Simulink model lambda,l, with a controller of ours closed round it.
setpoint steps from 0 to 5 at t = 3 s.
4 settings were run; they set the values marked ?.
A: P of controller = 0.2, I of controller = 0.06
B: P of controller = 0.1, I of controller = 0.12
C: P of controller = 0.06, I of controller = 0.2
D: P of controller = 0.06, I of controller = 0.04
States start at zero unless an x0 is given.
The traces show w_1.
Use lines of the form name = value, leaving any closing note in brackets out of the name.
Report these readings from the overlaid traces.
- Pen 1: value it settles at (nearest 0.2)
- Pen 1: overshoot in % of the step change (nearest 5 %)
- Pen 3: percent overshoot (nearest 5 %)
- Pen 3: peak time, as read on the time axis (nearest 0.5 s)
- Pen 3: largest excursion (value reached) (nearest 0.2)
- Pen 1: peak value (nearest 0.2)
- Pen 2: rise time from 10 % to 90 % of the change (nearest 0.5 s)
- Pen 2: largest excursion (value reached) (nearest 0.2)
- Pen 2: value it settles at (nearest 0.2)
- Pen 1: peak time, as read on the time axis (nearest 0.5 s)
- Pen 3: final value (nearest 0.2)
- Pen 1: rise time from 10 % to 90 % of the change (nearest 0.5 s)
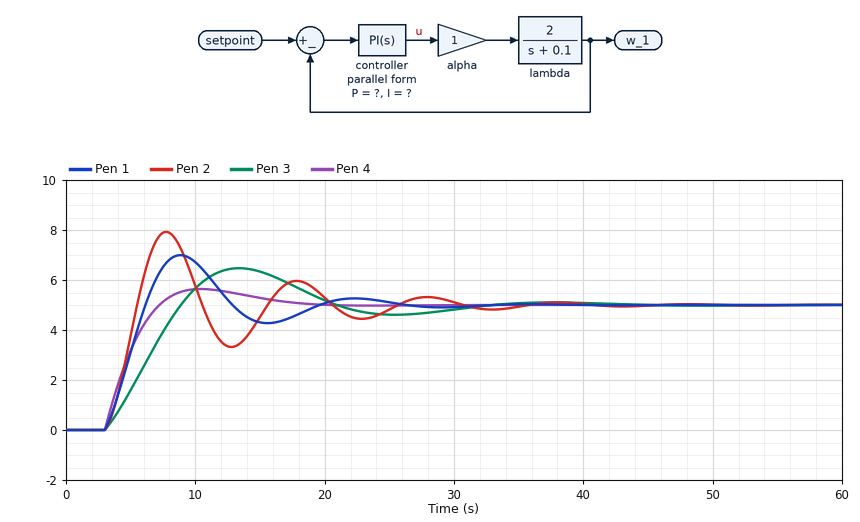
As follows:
Pen 1: value it settles at = 5.0
Pen 1: overshoot in % of the step change = 40 %
Pen 3: percent overshoot = 30 %
Pen 3: peak time, as read on the time axis = 13.5 s
Pen 3: largest excursion (value reached) = 6.4
Pen 1: peak value = 7.0
Pen 2: rise time from 10 % to 90 % of the change = 2.0 s
Pen 2: largest excursion (value reached) = 8.0
Pen 2: value it settles at = 5.0
Pen 1: peak time, as read on the time axis = 9.0 s
Pen 3: final value = 5.0
Pen 1: rise time from 10 % to 90 % of the change = 2.5 s
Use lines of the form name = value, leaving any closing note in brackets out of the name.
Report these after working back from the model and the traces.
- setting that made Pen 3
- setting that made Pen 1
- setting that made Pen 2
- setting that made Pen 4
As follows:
setting that made Pen 3 = D
setting that made Pen 1 = B
setting that made Pen 2 = C
setting that made Pen 4 = A
